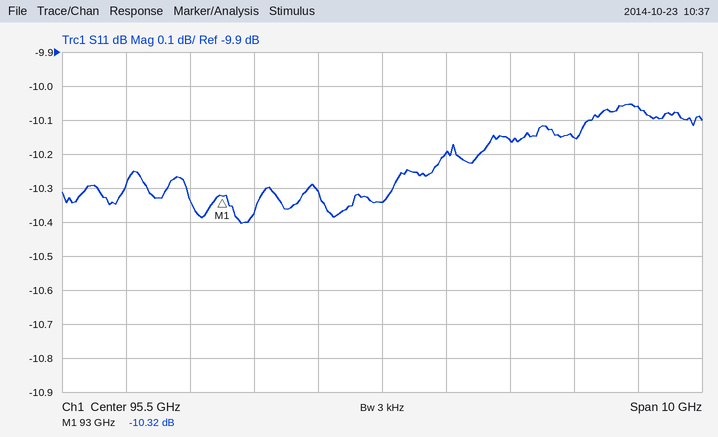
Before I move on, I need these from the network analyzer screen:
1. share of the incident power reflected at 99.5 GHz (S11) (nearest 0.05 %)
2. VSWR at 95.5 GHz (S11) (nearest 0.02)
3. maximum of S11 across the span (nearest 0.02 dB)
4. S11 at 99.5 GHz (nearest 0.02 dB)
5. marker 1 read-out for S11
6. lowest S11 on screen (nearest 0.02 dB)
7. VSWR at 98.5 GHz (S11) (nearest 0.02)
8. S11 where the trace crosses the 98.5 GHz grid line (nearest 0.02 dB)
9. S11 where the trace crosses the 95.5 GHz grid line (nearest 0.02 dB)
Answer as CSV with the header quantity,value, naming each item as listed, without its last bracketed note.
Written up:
quantity,value
share of the incident power reflected at 99.5 GHz (S11),9.85 %
VSWR at 95.5 GHz (S11),1.88
maximum of S11 across the span,-10.06 dB
S11 at 99.5 GHz,-10.06 dB
marker 1 read-out for S11,-10.32 dB
lowest S11 on screen,-10.40 dB
VSWR at 98.5 GHz (S11),1.90
S11 where the trace crosses the 98.5 GHz grid line,-10.16 dB
S11 where the trace crosses the 95.5 GHz grid line,-10.34 dB
